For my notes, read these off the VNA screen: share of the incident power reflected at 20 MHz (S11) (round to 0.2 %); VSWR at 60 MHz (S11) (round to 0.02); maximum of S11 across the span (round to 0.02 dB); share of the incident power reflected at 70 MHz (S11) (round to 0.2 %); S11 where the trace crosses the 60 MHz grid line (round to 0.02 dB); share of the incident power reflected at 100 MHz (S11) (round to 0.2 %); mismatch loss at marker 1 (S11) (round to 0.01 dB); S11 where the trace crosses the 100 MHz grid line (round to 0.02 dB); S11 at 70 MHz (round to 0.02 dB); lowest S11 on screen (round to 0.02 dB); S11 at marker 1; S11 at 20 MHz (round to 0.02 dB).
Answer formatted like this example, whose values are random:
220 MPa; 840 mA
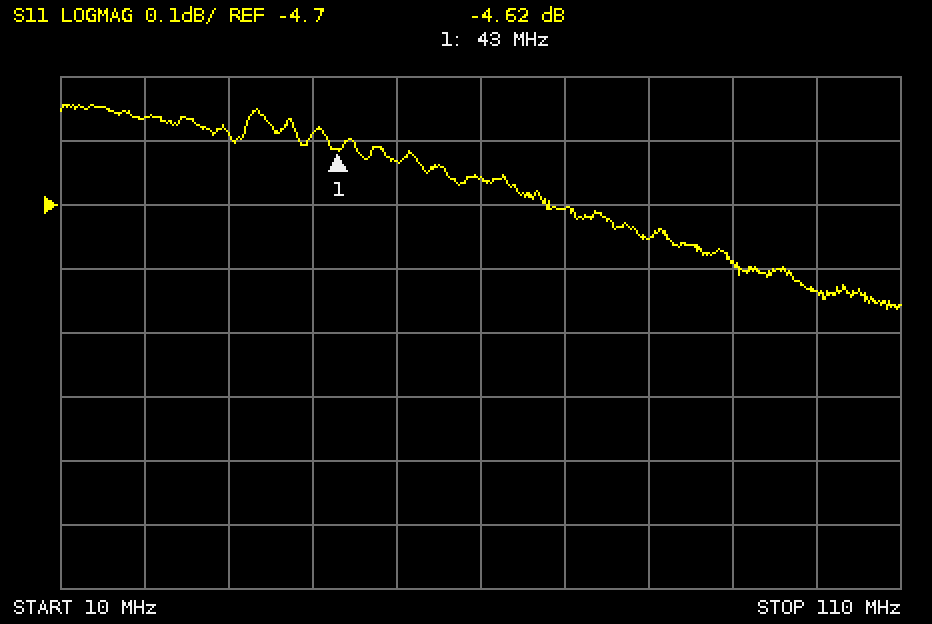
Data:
35.0 %; 3.82; -4.54 dB; 33.8 %; -4.66 dB; 32.8 %; 1.84 dB; -4.84 dB; -4.70 dB; -4.86 dB; -4.62 dB; -4.56 dB
